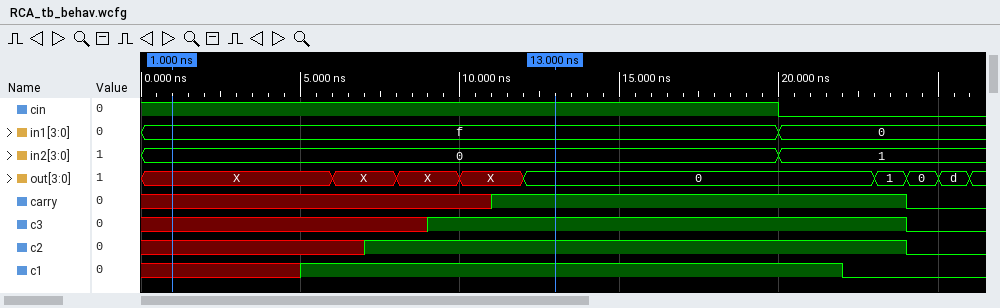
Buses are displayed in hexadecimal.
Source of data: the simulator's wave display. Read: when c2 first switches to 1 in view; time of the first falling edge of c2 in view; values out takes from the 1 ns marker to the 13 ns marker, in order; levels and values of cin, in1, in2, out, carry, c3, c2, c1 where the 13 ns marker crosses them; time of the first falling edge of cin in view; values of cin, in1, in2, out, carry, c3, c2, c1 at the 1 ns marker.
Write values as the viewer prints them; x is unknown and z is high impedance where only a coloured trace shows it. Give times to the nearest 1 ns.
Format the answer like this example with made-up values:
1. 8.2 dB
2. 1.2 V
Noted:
1. 7 ns
2. 24 ns
3. X, X, X, X, 0
4. cin=1, in1=f, in2=0, out=0, carry=1, c3=1, c2=1, c1=1
5. 20 ns
6. cin=1, in1=f, in2=0, out=X, carry=x, c3=x, c2=x, c1=x
